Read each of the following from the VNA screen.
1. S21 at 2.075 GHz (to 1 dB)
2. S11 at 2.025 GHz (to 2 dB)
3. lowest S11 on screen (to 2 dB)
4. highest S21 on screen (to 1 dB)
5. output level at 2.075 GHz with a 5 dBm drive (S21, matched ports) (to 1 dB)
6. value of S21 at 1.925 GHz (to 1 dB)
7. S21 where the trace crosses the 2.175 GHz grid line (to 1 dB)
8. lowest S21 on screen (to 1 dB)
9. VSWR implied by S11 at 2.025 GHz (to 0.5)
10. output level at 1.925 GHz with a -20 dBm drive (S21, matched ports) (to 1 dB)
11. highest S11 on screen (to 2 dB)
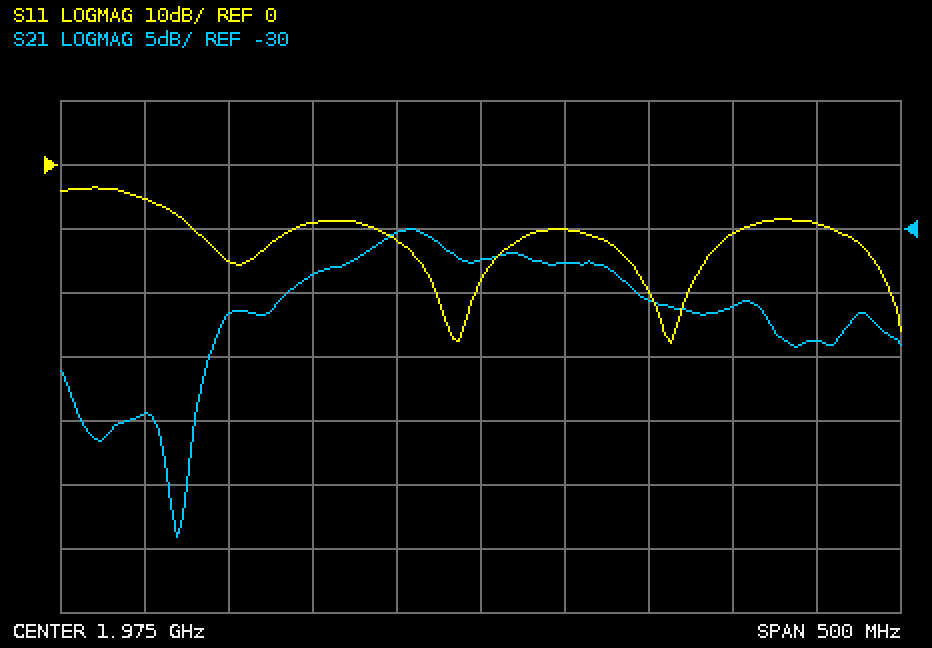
-36 dB
-10 dB
-28 dB
-30 dB
-31 dBm
-30 dB
-39 dB
-54 dB
2.0
-50 dBm
-4 dB
